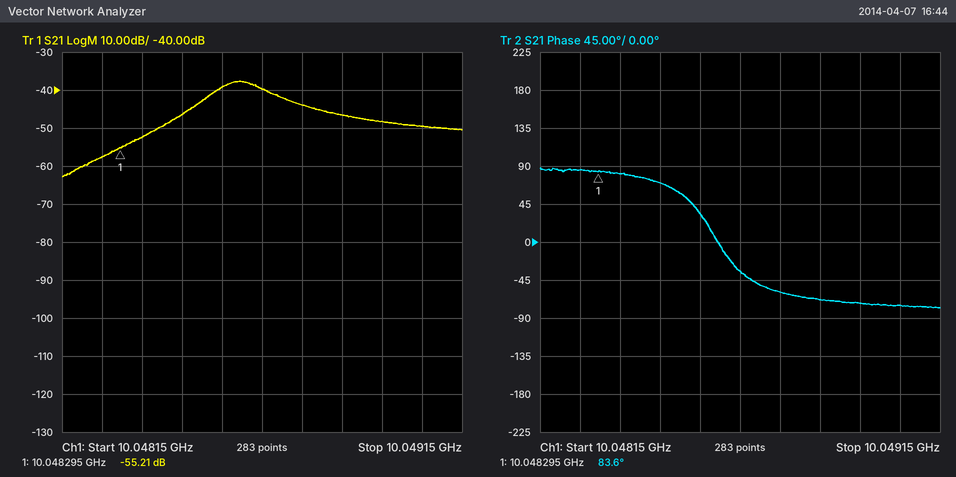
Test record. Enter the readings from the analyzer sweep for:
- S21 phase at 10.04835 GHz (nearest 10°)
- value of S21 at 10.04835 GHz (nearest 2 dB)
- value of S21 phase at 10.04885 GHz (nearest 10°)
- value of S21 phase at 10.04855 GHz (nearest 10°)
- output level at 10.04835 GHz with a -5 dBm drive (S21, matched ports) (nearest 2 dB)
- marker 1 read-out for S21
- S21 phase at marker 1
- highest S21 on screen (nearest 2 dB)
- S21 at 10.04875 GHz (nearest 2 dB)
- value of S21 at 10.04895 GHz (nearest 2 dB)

80°
-52 dB
-70°
30°
-58 dBm
-55.21 dB
83.6°
-38 dB
-44 dB
-48 dB
